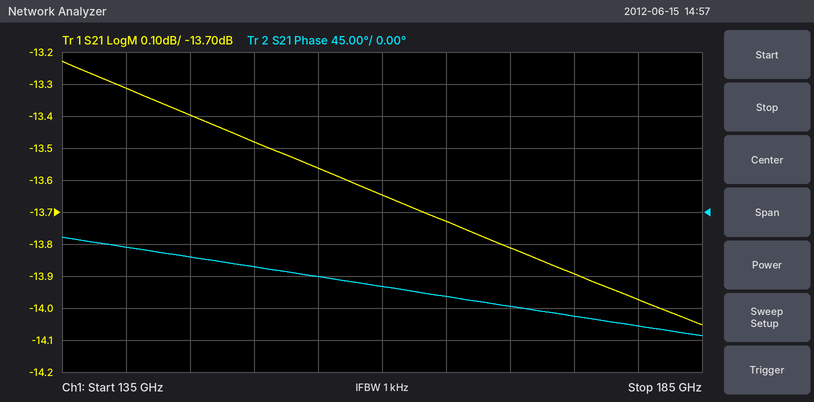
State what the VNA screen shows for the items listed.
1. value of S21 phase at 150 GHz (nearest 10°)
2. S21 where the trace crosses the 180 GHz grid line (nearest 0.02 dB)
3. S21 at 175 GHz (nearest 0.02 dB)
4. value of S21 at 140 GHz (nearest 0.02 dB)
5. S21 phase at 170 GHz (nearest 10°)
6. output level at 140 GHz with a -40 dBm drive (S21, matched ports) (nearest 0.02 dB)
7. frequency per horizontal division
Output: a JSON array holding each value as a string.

["-80°", "-13.98 dB", "-13.90 dB", "-13.32 dB", "-130°", "-53.32 dBm", "5 GHz"]
